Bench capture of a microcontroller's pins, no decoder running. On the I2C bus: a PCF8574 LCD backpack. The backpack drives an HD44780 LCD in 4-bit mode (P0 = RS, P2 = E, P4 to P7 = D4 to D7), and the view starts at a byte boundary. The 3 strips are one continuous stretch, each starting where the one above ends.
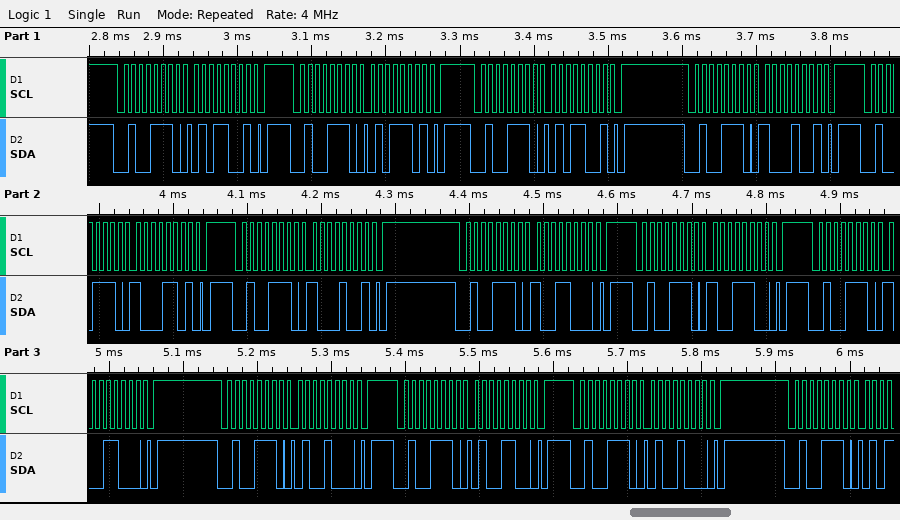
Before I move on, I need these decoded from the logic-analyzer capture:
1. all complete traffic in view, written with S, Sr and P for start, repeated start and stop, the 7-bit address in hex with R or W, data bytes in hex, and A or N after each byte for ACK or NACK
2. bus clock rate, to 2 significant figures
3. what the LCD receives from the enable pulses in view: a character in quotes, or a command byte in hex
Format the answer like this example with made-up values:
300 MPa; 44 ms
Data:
S 27W A 59 A P S 27W A 5D A P S 27W A 59 A P S 27W A 89 A P S 27W A 8D A P S 27W A 89 A P S 27W A 98 A P S 27W A 9C A P S 27W A 98 A P S 27W A 48 A P S 27W A 4C A P S 27W A 48 A P S 27W A; 100 kHz; 'X' 0x94
